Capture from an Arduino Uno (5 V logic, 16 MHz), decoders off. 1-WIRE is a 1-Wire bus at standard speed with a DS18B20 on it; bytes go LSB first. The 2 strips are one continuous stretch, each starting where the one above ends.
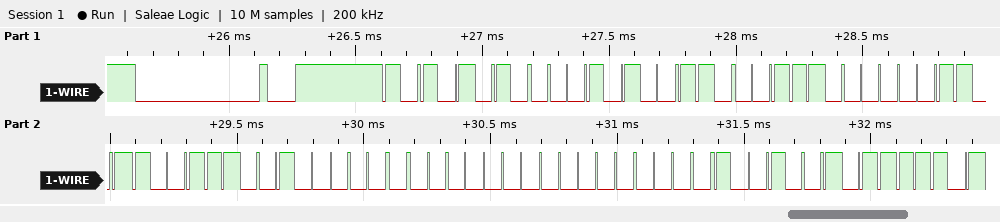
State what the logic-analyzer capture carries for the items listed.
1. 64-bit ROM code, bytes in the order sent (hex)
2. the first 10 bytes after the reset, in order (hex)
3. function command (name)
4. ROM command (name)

28 E3 C0 E6 04 00 00 92
55 28 E3 C0 E6 04 00 00 92 BE
Read Scratchpad
Match ROM
